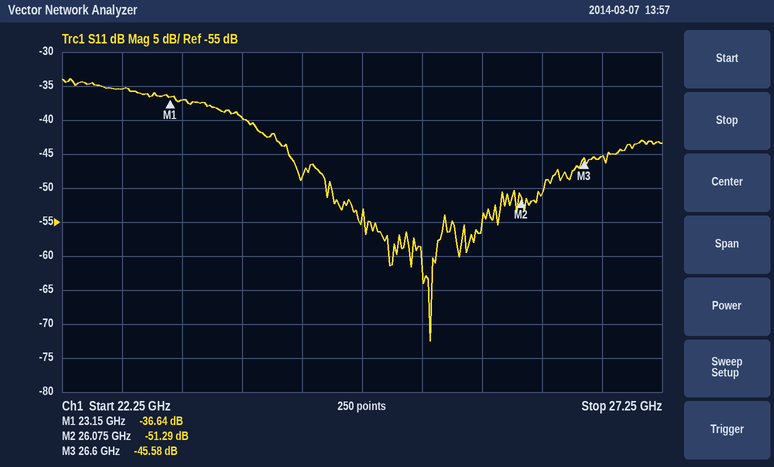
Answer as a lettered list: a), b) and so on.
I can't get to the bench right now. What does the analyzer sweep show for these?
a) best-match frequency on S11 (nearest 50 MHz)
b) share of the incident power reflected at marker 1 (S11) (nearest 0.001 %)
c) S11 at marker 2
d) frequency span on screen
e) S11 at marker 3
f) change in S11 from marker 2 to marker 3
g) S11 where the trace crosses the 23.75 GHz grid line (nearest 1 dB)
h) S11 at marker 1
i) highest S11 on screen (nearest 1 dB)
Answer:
a) 25.30 GHz
b) 0.022 %
c) -51.29 dB
d) 5 GHz
e) -45.58 dB
f) 5.71 dB
g) -40 dB
h) -36.64 dB
i) -34 dB
